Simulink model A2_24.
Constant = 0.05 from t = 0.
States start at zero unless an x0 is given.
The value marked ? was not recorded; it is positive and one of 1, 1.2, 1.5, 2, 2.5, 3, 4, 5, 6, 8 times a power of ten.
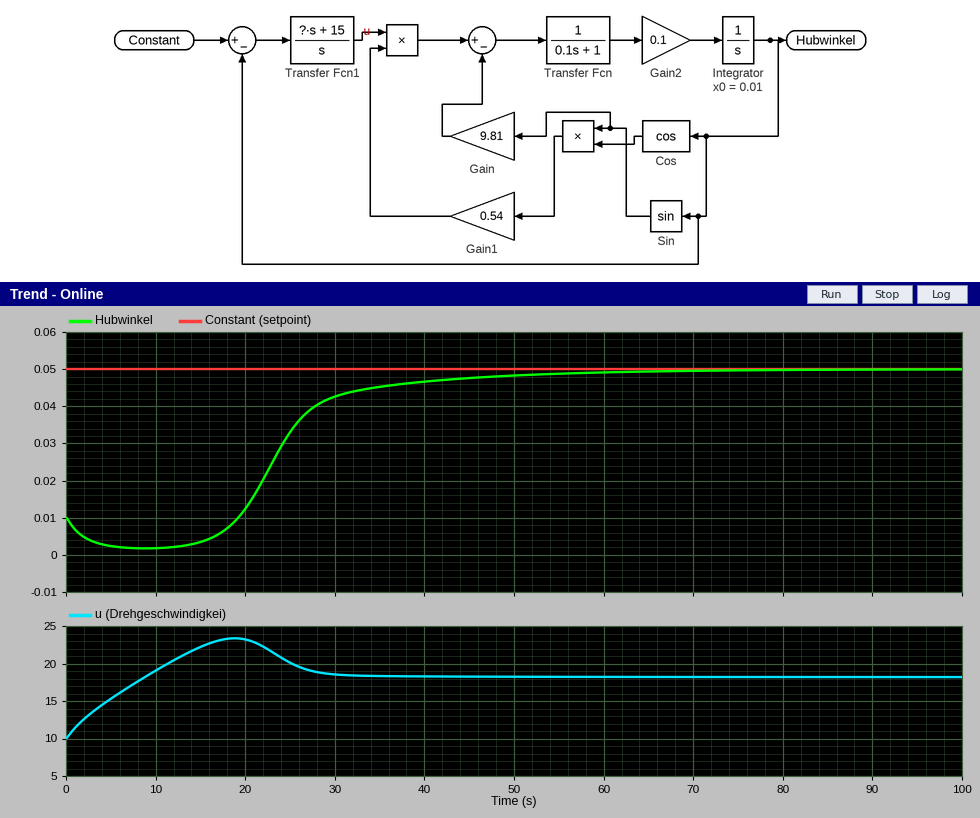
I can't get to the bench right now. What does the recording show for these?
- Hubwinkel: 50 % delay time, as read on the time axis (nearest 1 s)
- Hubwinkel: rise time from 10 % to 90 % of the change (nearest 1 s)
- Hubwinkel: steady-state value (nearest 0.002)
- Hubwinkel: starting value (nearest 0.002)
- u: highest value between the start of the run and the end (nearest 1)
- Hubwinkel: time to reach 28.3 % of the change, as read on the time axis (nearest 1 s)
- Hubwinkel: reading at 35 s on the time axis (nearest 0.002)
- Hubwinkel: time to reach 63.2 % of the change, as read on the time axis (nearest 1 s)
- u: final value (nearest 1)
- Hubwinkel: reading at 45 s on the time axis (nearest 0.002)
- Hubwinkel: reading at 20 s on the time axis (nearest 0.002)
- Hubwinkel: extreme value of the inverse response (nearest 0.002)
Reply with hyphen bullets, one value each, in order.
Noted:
- 24 s
- 17 s
- 0.050
- 0.010
- 23
- 22 s
- 0.046
- 26 s
- 18
- 0.048
- 0.012
- 0.002
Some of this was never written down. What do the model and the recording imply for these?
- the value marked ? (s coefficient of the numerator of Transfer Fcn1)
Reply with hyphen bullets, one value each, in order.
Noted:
- 250
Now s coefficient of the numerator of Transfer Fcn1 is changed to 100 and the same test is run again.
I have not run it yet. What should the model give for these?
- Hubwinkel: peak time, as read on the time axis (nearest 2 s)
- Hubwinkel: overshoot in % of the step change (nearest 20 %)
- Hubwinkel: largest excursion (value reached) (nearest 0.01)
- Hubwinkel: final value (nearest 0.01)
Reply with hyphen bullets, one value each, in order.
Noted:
- 44 s
- 180 %
- 0.12
- 0.05
